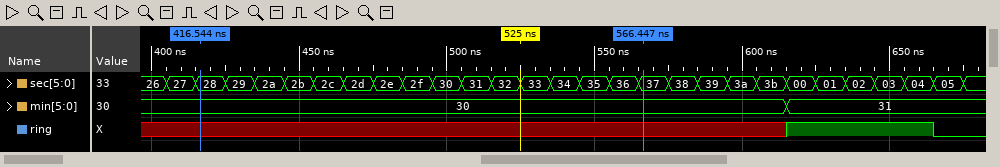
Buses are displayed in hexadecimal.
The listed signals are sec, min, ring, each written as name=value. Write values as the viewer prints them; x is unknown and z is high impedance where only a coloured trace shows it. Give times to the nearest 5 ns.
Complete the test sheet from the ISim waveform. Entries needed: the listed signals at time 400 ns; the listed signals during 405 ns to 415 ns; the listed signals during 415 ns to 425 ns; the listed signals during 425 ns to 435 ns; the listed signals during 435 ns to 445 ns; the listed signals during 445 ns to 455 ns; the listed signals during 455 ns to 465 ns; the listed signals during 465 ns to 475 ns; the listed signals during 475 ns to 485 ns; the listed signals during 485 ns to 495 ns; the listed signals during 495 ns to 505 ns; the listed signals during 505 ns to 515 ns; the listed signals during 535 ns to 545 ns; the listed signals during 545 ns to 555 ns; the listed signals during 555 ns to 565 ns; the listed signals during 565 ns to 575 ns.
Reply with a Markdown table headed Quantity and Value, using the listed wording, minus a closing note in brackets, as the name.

| Quantity | Value |
|---|---|
| the listed signals at time 400 ns | sec=26, min=30, ring=x |
| the listed signals during 405 ns to 415 ns | sec=27, min=30, ring=x |
| the listed signals during 415 ns to 425 ns | sec=28, min=30, ring=x |
| the listed signals during 425 ns to 435 ns | sec=29, min=30, ring=x |
| the listed signals during 435 ns to 445 ns | sec=2a, min=30, ring=x |
| the listed signals during 445 ns to 455 ns | sec=2b, min=30, ring=x |
| the listed signals during 455 ns to 465 ns | sec=2c, min=30, ring=x |
| the listed signals during 465 ns to 475 ns | sec=2d, min=30, ring=x |
| the listed signals during 475 ns to 485 ns | sec=2e, min=30, ring=x |
| the listed signals during 485 ns to 495 ns | sec=2f, min=30, ring=x |
| the listed signals during 495 ns to 505 ns | sec=30, min=30, ring=x |
| the listed signals during 505 ns to 515 ns | sec=31, min=30, ring=x |
| the listed signals during 535 ns to 545 ns | sec=34, min=30, ring=x |
| the listed signals during 545 ns to 555 ns | sec=35, min=30, ring=x |
| the listed signals during 555 ns to 565 ns | sec=36, min=30, ring=x |
| the listed signals during 565 ns to 575 ns | sec=37, min=30, ring=x |
